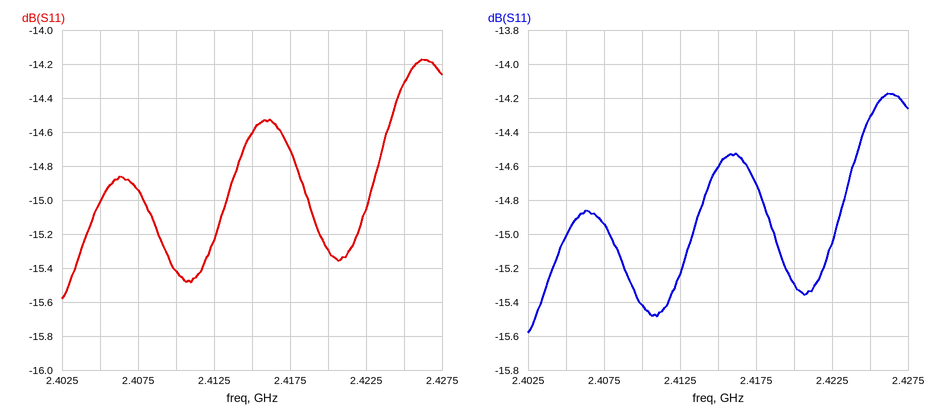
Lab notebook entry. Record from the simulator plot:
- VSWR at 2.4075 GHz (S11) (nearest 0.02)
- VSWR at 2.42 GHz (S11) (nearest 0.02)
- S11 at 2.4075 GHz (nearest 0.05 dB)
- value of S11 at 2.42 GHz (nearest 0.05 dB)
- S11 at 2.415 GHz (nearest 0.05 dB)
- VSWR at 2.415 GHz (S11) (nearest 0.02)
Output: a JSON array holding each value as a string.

["1.44", "1.42", "-14.95 dB", "-15.30 dB", "-14.60 dB", "1.46"]
